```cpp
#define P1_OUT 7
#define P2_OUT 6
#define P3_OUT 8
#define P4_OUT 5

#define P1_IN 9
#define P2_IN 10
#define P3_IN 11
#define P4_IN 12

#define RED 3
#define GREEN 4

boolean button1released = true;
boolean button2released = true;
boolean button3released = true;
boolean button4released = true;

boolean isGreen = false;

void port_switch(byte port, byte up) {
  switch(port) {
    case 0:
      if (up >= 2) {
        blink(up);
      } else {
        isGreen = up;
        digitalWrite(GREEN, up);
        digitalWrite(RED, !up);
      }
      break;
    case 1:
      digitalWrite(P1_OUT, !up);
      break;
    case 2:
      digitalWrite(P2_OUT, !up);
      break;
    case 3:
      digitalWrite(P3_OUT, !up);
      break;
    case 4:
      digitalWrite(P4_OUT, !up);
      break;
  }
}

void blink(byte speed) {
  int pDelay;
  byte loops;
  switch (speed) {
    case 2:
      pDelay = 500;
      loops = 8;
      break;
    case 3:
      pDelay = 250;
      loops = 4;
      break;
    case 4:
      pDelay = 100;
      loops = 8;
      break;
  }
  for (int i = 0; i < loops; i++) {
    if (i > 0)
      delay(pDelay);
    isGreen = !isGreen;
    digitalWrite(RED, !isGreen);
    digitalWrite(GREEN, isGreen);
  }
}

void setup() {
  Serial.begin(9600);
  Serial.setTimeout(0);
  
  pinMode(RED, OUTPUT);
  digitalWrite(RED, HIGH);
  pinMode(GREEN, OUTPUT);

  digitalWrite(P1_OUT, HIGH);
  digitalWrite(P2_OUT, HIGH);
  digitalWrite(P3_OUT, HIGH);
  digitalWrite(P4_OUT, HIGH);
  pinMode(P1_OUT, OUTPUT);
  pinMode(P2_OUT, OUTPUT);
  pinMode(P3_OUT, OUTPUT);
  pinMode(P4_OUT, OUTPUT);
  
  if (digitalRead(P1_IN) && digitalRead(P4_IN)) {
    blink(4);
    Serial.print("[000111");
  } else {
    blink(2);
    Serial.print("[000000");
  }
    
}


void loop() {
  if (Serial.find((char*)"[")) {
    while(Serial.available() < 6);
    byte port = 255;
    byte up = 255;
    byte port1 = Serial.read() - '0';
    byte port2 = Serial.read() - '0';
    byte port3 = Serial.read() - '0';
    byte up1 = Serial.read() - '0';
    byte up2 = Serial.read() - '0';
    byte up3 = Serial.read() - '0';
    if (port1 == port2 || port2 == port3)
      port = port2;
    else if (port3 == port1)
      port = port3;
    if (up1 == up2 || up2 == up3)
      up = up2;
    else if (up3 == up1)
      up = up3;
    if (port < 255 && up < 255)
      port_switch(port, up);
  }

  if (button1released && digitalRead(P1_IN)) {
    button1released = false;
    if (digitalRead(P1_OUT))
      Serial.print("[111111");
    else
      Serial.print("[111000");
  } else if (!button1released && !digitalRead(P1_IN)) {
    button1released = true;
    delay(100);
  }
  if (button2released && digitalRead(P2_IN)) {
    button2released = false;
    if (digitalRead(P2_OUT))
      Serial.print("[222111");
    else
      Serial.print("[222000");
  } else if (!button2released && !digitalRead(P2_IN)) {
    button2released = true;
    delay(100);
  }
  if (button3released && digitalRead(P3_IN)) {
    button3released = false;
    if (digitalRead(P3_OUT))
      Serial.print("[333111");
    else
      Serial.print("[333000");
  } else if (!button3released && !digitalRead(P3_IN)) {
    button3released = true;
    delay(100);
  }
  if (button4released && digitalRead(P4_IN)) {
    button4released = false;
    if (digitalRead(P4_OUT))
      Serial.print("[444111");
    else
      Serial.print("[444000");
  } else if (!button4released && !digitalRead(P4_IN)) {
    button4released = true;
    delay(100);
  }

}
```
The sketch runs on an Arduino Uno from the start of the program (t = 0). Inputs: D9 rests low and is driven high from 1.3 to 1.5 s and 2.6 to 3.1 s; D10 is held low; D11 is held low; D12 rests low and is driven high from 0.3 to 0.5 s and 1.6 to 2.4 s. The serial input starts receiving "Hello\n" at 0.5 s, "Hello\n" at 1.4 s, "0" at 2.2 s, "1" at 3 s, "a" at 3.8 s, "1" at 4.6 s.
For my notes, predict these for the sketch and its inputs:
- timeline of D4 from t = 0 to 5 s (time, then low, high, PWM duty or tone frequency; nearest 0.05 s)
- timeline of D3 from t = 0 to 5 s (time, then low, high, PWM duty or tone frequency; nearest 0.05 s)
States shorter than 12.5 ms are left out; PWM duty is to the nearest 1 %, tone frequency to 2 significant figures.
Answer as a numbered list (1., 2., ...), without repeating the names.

1. 0 s high; 0.5 s low; 1 s high; 1.5 s low; 2 s high; 2.5 s low; 3 s high; 3.5 s low
2. 0 s low; 0.5 s high; 1 s low; 1.5 s high; 2 s low; 2.5 s high; 3 s low; 3.5 s high
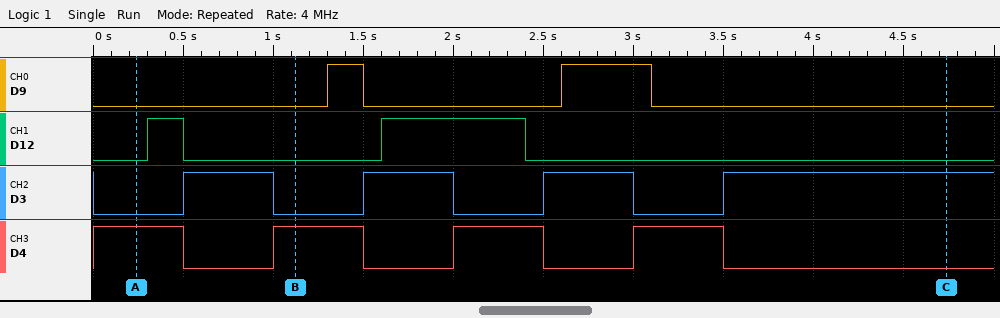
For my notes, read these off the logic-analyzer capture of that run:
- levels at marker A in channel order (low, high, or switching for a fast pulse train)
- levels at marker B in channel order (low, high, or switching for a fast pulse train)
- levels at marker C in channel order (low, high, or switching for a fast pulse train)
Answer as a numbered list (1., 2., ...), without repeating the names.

1. D9 low, D12 low, D3 low, D4 high
2. D9 low, D12 low, D3 low, D4 high
3. D9 low, D12 low, D3 high, D4 low
